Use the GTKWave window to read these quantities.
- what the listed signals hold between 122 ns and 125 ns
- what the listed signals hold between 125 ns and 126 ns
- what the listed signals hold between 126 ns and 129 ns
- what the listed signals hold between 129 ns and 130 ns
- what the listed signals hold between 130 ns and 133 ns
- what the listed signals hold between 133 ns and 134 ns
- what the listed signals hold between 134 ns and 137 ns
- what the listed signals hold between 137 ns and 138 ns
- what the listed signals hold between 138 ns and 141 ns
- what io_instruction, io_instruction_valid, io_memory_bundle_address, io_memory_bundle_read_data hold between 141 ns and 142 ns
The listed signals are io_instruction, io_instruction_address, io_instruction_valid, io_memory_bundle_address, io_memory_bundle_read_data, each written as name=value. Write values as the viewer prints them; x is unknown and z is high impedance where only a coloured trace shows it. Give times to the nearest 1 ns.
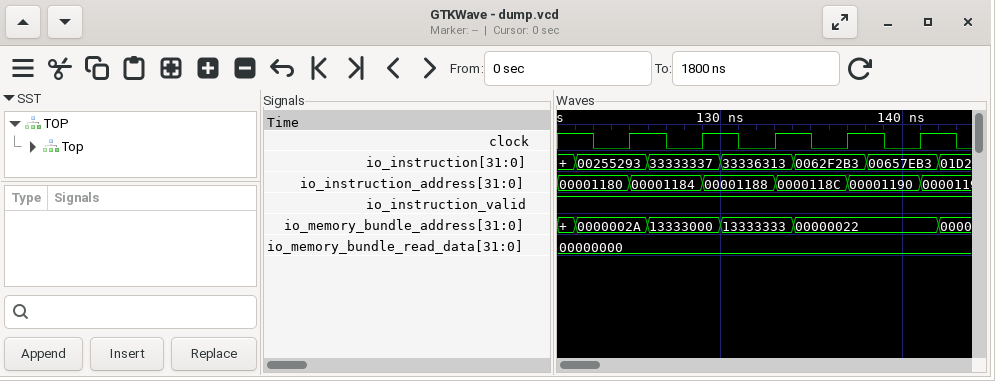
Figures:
io_instruction=00255293, io_instruction_address=00001180, io_instruction_valid=1, io_memory_bundle_address=0000002A, io_memory_bundle_read_data=00000000
io_instruction=00255293, io_instruction_address=00001184, io_instruction_valid=1, io_memory_bundle_address=0000002A, io_memory_bundle_read_data=00000000
io_instruction=33333337, io_instruction_address=00001184, io_instruction_valid=1, io_memory_bundle_address=13333000, io_memory_bundle_read_data=00000000
io_instruction=33333337, io_instruction_address=00001188, io_instruction_valid=1, io_memory_bundle_address=13333000, io_memory_bundle_read_data=00000000
io_instruction=33336313, io_instruction_address=00001188, io_instruction_valid=1, io_memory_bundle_address=13333333, io_memory_bundle_read_data=00000000
io_instruction=33336313, io_instruction_address=0000118C, io_instruction_valid=1, io_memory_bundle_address=13333333, io_memory_bundle_read_data=00000000
io_instruction=0062F2B3, io_instruction_address=0000118C, io_instruction_valid=1, io_memory_bundle_address=00000022, io_memory_bundle_read_data=00000000
io_instruction=0062F2B3, io_instruction_address=00001190, io_instruction_valid=1, io_memory_bundle_address=00000022, io_memory_bundle_read_data=00000000
io_instruction=00657EB3, io_instruction_address=00001190, io_instruction_valid=1, io_memory_bundle_address=00000022, io_memory_bundle_read_data=00000000
io_instruction=00657EB3, io_instruction_valid=1, io_memory_bundle_address=00000022, io_memory_bundle_read_data=00000000
